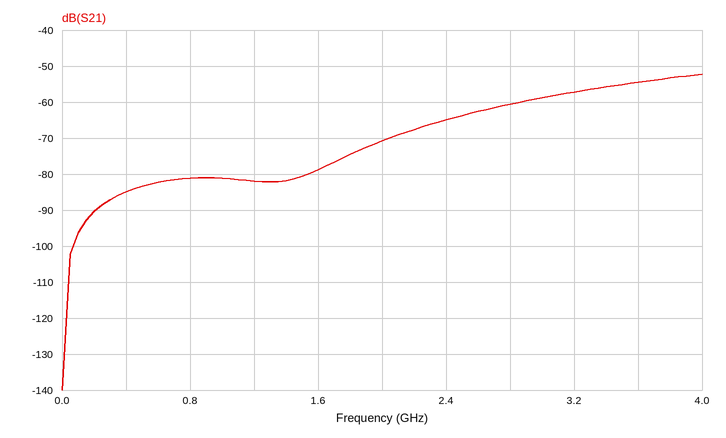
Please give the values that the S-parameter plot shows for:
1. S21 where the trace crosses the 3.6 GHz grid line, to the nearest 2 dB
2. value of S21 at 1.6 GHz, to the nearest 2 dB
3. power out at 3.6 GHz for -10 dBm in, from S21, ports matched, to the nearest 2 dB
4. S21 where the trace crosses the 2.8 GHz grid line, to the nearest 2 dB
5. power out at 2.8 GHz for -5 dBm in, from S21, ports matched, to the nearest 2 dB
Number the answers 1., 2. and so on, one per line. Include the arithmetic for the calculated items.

1. -54 dB
2. -78 dB
3. -10 dBm + (-54 dB) = -64 dBm
4. -60 dB
5. -5 dBm + (-60 dB) = -66 dBm
